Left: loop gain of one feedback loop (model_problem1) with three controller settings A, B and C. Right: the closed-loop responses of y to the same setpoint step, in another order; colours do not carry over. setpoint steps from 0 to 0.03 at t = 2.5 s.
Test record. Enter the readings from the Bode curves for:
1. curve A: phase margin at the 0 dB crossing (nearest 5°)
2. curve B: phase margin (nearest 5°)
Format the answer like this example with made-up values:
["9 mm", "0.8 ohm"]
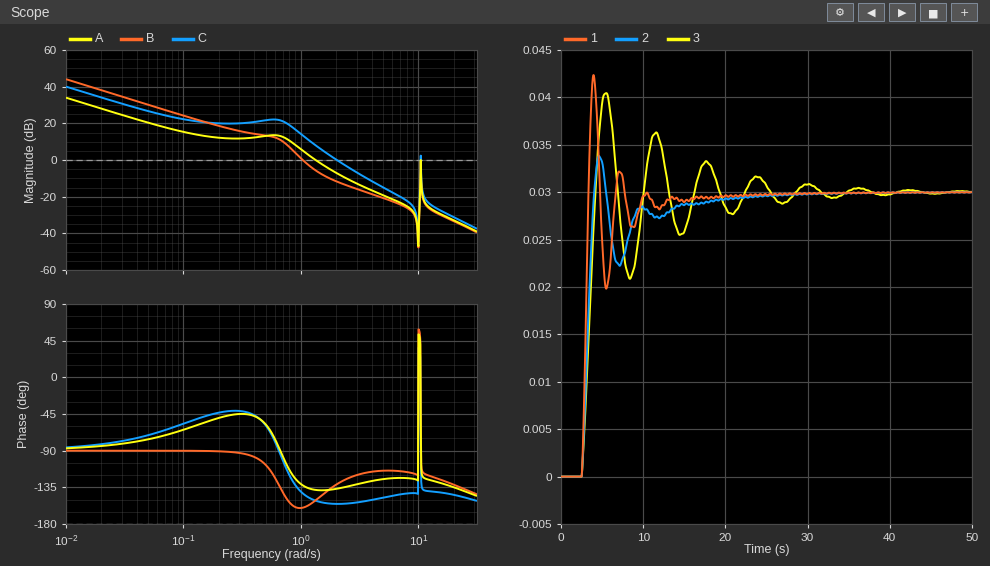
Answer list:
["40°", "20°"]
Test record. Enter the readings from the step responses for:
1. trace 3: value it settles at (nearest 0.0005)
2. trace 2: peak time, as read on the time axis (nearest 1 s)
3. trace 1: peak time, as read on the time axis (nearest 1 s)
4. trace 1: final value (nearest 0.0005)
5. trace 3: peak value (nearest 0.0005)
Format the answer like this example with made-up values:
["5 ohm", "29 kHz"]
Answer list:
["0.0300", "5 s", "4 s", "0.0300", "0.0405"]
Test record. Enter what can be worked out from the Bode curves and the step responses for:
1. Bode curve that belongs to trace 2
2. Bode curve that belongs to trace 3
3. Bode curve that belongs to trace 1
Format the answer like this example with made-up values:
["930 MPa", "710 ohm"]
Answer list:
["A", "B", "C"]
